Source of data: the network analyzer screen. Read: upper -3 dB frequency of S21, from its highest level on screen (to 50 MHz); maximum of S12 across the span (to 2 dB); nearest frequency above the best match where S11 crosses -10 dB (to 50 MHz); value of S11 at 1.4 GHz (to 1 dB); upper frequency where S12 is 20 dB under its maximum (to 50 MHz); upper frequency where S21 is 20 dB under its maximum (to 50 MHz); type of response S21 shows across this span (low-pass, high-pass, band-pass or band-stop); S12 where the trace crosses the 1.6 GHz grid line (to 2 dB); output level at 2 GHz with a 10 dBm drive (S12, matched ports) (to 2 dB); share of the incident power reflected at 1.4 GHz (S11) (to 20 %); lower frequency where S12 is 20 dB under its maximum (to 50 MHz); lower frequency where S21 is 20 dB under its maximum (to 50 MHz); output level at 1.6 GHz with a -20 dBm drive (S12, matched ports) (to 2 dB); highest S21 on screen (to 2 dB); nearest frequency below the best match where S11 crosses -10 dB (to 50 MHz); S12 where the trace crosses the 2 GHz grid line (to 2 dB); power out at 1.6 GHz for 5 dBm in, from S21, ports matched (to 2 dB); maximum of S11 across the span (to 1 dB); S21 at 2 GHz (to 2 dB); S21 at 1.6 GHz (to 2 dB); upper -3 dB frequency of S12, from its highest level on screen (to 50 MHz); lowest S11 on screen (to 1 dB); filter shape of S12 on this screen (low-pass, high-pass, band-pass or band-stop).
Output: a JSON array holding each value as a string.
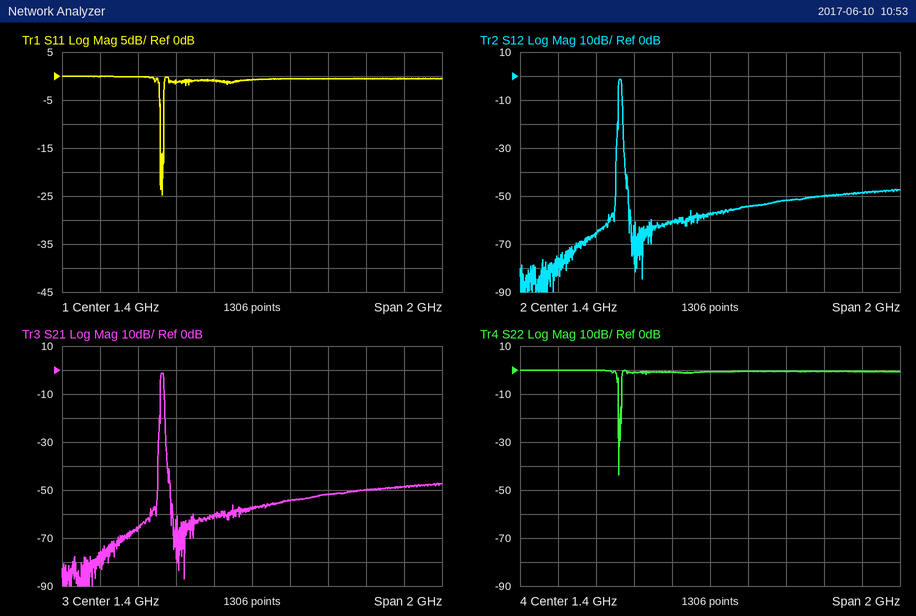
["950 MHz", "-2 dB", "950 MHz", "-1 dB", "950 MHz", "950 MHz", "band-pass", "-54 dB", "-40 dBm", "80 %", "900 MHz", "900 MHz", "-74 dBm", "-2 dB", "900 MHz", "-50 dB", "-50 dBm", "0 dB", "-50 dB", "-54 dB", "950 MHz", "-25 dB", "band-pass"]
